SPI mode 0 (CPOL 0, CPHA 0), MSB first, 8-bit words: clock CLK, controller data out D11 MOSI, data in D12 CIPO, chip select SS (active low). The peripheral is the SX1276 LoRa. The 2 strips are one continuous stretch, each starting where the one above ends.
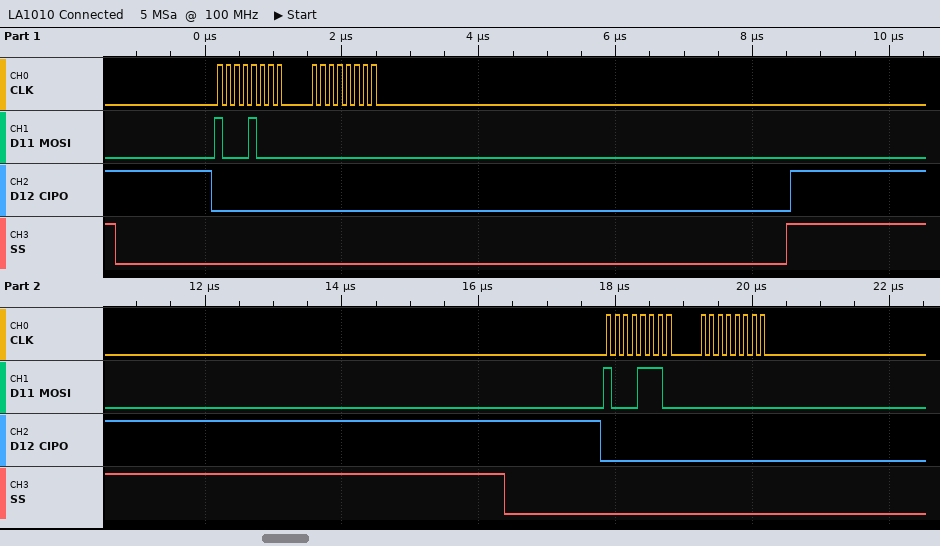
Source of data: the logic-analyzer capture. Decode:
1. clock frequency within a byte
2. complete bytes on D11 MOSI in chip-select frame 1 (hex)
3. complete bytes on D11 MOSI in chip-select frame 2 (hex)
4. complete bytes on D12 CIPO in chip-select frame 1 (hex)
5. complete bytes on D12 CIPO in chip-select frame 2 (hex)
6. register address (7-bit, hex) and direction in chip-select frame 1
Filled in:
8 MHz
88 00
8E 00
00 00
00 00
0x08 write
